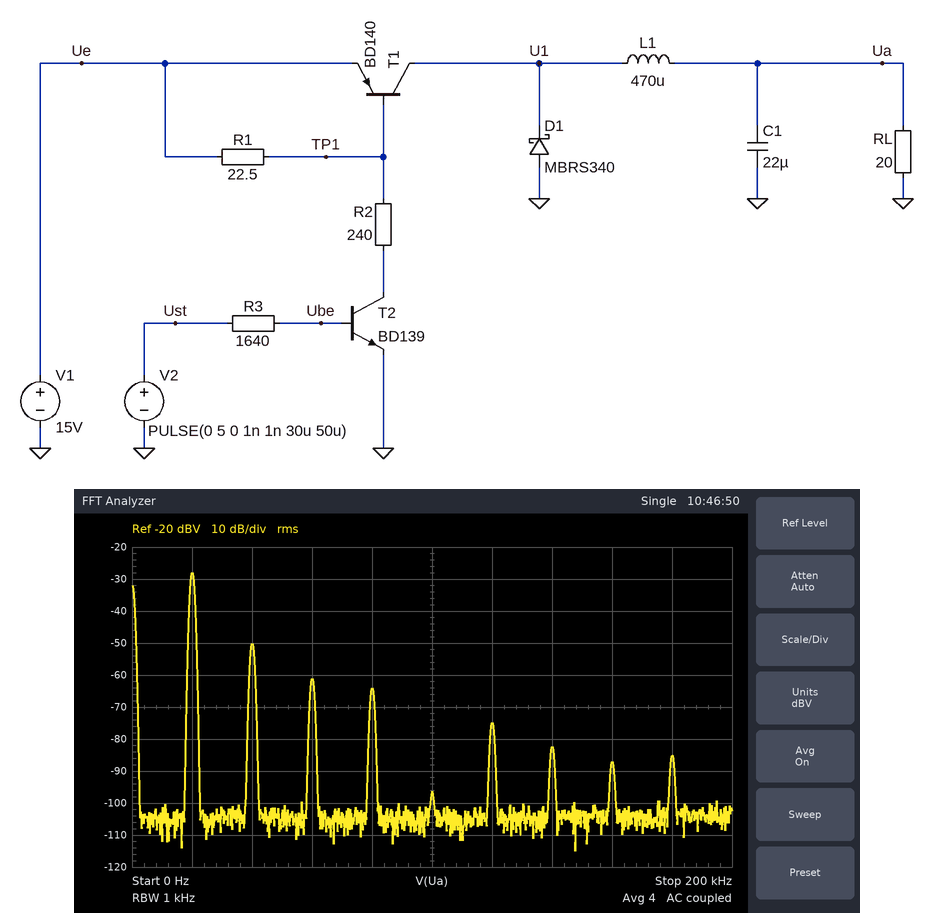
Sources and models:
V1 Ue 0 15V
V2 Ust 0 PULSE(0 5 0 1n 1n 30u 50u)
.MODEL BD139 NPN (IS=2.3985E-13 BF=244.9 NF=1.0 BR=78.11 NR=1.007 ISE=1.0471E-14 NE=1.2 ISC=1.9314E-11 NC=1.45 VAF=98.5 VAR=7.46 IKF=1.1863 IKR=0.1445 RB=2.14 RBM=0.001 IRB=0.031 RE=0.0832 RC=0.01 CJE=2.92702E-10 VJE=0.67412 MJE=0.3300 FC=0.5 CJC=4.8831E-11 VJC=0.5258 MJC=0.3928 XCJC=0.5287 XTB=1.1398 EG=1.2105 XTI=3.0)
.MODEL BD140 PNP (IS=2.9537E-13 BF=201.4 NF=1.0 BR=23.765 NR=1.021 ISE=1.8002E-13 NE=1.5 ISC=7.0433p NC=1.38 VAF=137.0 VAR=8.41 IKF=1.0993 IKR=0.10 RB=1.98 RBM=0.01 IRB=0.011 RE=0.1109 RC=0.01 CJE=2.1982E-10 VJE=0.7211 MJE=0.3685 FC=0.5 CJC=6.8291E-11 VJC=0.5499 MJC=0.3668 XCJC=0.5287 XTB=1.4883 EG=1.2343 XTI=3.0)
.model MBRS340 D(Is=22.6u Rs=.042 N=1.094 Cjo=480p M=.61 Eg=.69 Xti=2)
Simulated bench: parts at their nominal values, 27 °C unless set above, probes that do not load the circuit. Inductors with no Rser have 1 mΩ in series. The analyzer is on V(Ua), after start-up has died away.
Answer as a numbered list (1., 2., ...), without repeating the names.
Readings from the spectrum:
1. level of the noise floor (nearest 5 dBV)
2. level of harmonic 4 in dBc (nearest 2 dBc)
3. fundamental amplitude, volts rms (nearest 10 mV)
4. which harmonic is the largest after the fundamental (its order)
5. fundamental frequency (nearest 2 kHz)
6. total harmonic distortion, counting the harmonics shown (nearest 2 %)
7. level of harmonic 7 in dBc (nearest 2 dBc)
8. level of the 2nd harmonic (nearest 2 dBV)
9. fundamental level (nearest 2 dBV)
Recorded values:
1. -105 dBV
2. -36 dBc
3. 40 mV
4. 2
5. 20 kHz
6. 8 %
7. -54 dBc
8. -50 dBV
9. -28 dBV
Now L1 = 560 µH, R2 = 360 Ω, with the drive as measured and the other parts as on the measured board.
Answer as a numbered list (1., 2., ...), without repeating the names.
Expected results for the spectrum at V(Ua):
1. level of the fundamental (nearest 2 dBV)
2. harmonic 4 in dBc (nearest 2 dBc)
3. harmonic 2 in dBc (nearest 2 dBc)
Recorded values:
1. -30 dBV
2. -38 dBc
3. -30 dBc
